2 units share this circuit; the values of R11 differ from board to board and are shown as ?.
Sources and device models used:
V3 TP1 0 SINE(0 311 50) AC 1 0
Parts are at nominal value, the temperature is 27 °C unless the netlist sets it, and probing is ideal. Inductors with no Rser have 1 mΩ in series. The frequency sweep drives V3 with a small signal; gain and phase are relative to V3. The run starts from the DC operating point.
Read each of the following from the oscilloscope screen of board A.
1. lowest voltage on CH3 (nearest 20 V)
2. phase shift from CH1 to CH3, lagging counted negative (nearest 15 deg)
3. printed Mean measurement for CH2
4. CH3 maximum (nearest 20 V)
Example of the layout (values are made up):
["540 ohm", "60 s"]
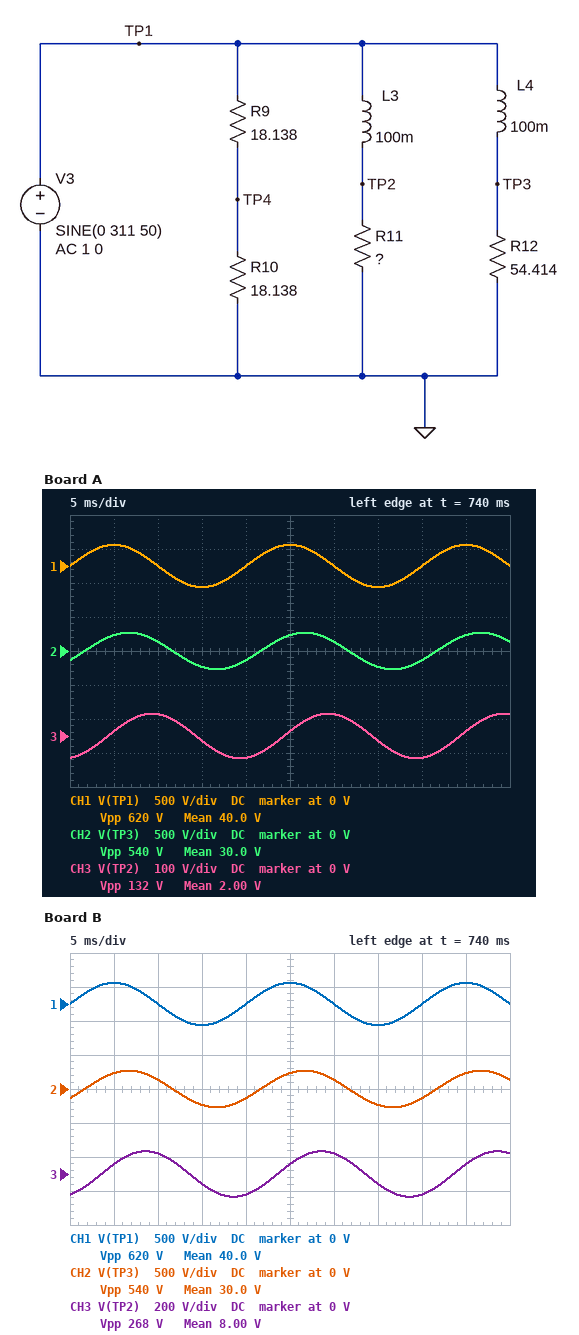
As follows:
["-60 V", "-75 deg", "30.0 V", "60 V"]
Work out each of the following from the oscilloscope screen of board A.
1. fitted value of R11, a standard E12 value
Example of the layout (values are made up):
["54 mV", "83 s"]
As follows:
["6.8 Ω"]
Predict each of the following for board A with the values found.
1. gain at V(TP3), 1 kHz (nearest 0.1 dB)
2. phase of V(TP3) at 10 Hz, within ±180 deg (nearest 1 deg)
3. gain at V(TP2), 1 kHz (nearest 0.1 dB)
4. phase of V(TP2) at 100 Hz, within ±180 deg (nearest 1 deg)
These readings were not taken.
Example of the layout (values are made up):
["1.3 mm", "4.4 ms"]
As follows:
["-21.3 dB", "-7 deg", "-39.3 dB", "-84 deg"]
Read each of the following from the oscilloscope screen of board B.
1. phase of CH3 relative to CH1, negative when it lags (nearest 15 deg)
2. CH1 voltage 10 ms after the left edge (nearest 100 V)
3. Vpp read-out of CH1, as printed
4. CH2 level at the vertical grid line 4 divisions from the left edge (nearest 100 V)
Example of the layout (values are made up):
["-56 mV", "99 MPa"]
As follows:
["-60 deg", "0 V", "620 V", "-100 V"]
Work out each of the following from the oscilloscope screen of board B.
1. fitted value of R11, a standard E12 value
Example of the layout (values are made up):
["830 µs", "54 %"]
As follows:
["15 Ω"]
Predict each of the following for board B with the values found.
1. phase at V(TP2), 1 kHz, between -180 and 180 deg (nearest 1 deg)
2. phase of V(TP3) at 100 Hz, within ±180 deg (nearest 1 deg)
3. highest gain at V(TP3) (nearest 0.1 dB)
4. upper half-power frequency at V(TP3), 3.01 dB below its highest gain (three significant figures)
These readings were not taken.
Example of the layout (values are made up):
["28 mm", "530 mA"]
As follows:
["-89 deg", "-49 deg", "0 dB", "86.6 Hz"]
